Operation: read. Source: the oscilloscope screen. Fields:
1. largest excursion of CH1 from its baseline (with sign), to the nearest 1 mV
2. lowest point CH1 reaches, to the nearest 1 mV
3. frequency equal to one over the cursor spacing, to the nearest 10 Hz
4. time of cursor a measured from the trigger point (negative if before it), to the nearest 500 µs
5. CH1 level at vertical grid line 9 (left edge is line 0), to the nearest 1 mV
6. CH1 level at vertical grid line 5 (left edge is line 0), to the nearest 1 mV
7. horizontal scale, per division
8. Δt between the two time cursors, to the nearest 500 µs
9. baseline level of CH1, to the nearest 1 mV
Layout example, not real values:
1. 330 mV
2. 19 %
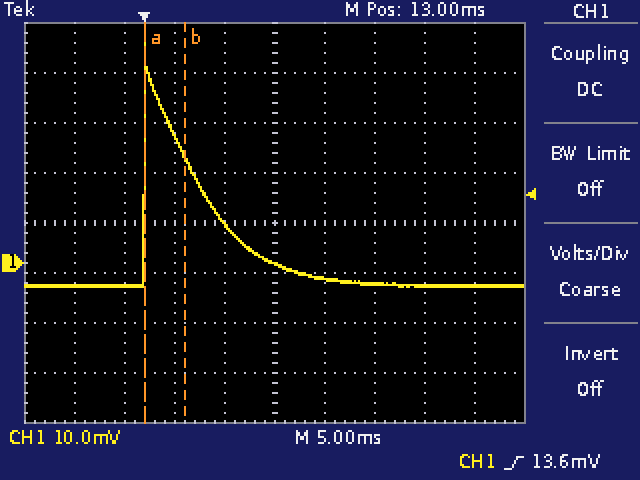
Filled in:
1. +49 mV
2. -5 mV
3. 250 Hz
4. 0.0 ms
5. -5 mV
6. 0 mV
7. 5 ms
8. 4.0 ms
9. -5 mV
